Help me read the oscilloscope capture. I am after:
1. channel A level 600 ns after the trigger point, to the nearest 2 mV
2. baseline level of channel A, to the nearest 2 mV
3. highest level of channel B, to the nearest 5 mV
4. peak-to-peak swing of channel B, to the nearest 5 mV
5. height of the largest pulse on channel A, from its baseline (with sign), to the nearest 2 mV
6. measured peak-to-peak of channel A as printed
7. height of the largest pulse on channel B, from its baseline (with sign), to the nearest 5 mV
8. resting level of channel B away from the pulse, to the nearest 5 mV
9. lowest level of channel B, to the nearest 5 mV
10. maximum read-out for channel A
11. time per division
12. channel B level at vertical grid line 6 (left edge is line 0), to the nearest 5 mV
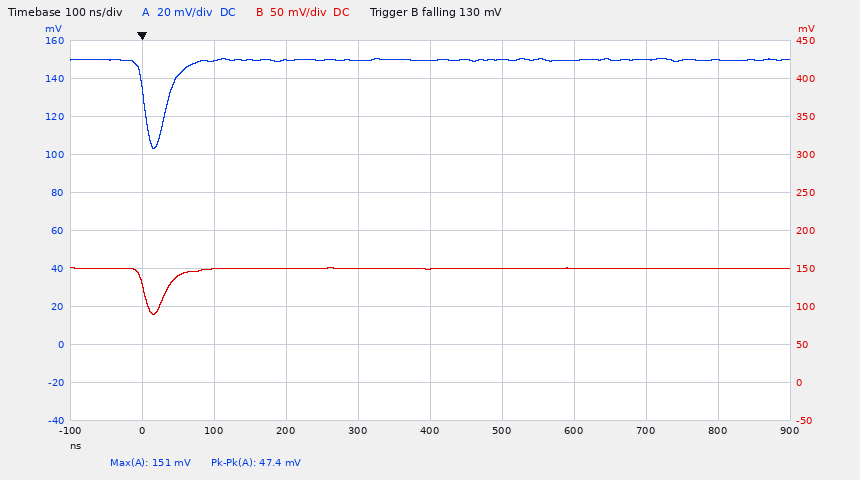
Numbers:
150 mV
150 mV
150 mV
60 mV
-46 mV
47.4 mV
-60 mV
150 mV
90 mV
151 mV
100 ns
150 mV
